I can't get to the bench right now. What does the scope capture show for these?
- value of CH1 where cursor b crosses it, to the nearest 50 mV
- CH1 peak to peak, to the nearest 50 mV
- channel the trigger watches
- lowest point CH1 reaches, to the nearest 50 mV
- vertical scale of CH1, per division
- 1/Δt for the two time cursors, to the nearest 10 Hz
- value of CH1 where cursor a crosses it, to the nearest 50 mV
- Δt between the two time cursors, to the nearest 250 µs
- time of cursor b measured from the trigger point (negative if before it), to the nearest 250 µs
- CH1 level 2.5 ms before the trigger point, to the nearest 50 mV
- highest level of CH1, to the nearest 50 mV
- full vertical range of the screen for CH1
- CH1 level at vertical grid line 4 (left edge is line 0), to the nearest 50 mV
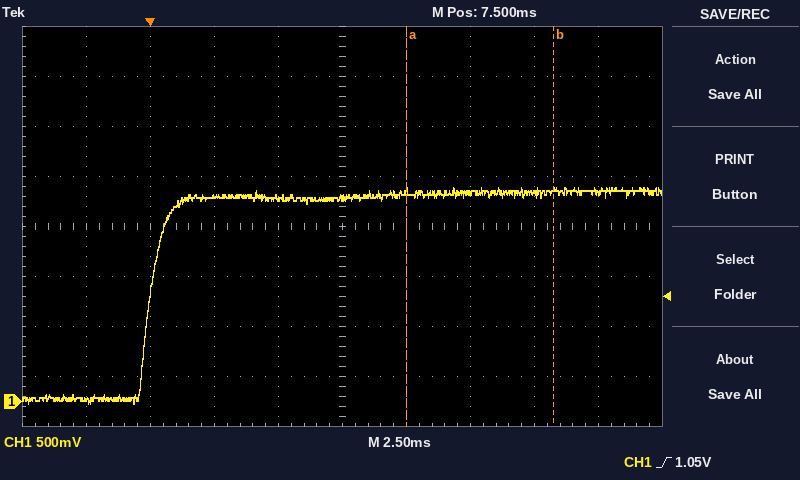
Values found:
2.10 V
2.15 V
CH1
0 mV
500 mV
170 Hz
2.10 V
5.75 ms
+15.75 ms
0 mV
2.15 V
4 V
2.05 V
